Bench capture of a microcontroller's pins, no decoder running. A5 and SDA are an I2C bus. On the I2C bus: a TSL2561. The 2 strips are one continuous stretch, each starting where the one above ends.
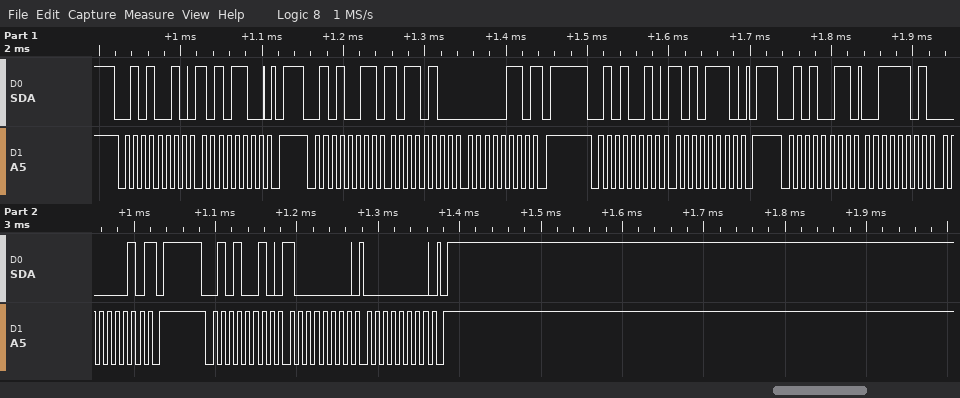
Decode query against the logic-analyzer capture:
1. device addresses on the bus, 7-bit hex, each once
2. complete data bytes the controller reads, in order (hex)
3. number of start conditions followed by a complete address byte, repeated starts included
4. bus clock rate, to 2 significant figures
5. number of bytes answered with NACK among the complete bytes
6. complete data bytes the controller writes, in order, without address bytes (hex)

0x29
B4 06 3D 02
5
100 kHz
2
AC AE 80 00
